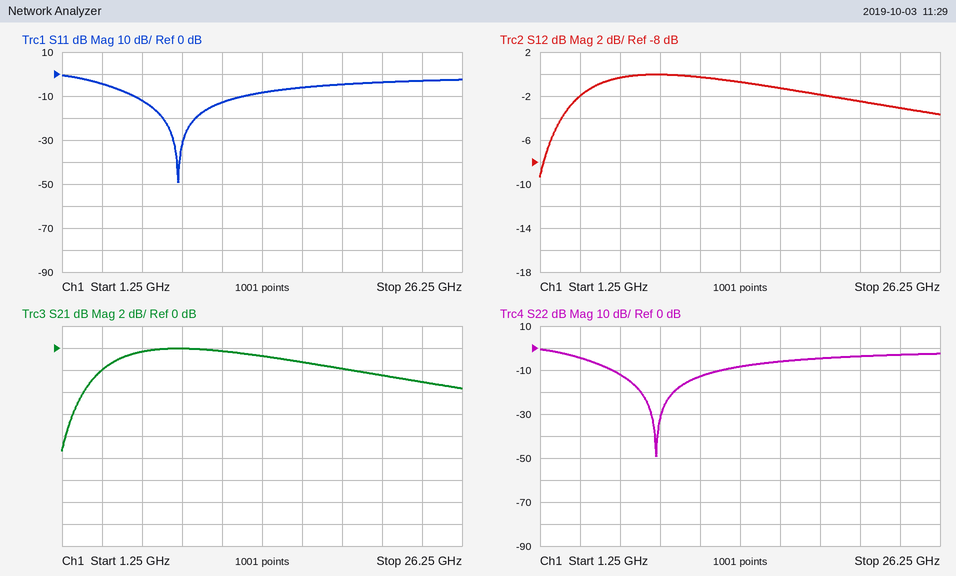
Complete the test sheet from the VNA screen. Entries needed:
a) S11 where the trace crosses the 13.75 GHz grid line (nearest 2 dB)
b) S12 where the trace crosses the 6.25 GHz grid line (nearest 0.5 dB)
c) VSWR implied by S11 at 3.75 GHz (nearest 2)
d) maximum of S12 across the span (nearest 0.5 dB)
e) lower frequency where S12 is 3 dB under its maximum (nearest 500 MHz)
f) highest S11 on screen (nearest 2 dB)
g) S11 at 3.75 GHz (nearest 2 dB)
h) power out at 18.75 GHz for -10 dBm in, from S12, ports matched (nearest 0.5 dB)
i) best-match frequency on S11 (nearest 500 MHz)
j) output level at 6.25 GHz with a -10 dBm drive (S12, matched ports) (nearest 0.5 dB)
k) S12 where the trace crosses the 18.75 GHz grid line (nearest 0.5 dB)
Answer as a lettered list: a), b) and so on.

a) -8 dB
b) -0.5 dB
c) 4
d) 0.0 dB
e) 3.0 GHz
f) 0 dB
g) -4 dB
h) -12.0 dBm
i) 8.5 GHz
j) -10.5 dBm
k) -2.0 dB
